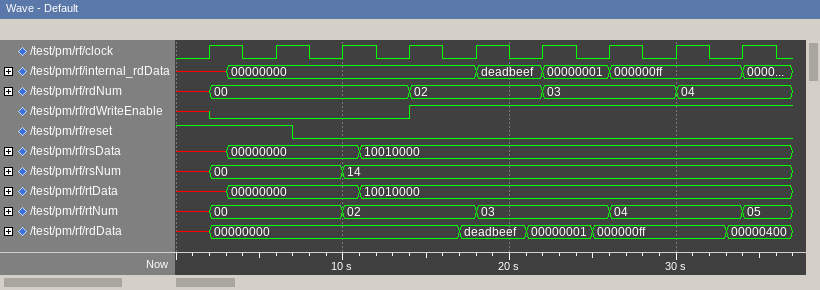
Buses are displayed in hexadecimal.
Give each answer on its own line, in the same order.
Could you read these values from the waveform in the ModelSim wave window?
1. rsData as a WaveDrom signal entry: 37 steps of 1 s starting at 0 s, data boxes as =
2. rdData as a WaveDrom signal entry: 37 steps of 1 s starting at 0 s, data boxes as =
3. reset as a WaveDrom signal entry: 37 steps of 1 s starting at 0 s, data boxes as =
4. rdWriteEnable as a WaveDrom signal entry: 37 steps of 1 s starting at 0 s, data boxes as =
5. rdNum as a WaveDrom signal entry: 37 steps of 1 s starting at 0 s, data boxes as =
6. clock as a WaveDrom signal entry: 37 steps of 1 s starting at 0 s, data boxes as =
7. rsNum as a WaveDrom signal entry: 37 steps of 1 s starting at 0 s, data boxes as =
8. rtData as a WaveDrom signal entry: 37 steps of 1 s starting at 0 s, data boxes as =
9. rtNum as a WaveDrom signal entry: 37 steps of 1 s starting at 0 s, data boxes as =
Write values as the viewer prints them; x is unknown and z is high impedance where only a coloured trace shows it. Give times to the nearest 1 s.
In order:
{name: 'rsData', wave: 'x..=.......=.........................', data: '00000000 10010000'}
{name: 'rdData', wave: 'x.=..............=...=...=.......=...', data: '00000000 deadbeef 00000001 000000ff 00000400'}
{name: 'reset', wave: '1......0.............................'}
{name: 'rdWriteEnable', wave: 'x.0...........1......................'}
{name: 'rdNum', wave: 'x.=...........=.......=.......=......', data: '00 02 03 04'}
{name: 'clock', wave: '0.1.0.1.0.1.0.1.0.1.0.1.0.1.0.1.0.1.0'}
{name: 'rsNum', wave: 'x.=.......=..........................', data: '00 14'}
{name: 'rtData', wave: 'x..=.......=.........................', data: '00000000 10010000'}
{name: 'rtNum', wave: 'x.=.......=.......=.......=.......=..', data: '00 02 03 04 05'}
